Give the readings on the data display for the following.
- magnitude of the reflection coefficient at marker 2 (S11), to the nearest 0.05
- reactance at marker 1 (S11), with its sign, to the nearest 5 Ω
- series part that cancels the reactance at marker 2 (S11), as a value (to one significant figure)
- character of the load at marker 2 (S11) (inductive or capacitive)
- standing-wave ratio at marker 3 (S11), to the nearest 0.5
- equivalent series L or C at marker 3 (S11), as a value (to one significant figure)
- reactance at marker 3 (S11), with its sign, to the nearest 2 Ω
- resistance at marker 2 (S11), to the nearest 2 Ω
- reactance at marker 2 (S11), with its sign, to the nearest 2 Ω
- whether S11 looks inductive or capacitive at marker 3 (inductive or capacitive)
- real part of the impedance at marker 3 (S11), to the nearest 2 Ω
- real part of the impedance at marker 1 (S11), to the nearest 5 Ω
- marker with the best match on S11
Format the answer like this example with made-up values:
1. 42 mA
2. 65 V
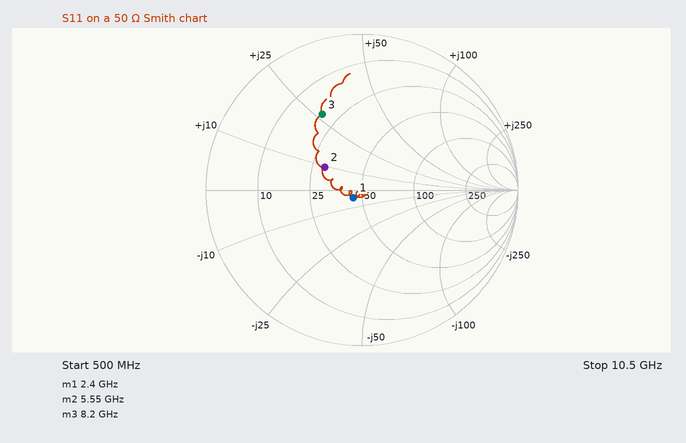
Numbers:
1. 0.30
2. -5 Ω
3. 3 pF
4. inductive
5. 3.5
6. 500 pH
7. +26 Ω
8. 30 Ω
9. +10 Ω
10. inductive
11. 20 Ω
12. 45 Ω
13. marker 1
